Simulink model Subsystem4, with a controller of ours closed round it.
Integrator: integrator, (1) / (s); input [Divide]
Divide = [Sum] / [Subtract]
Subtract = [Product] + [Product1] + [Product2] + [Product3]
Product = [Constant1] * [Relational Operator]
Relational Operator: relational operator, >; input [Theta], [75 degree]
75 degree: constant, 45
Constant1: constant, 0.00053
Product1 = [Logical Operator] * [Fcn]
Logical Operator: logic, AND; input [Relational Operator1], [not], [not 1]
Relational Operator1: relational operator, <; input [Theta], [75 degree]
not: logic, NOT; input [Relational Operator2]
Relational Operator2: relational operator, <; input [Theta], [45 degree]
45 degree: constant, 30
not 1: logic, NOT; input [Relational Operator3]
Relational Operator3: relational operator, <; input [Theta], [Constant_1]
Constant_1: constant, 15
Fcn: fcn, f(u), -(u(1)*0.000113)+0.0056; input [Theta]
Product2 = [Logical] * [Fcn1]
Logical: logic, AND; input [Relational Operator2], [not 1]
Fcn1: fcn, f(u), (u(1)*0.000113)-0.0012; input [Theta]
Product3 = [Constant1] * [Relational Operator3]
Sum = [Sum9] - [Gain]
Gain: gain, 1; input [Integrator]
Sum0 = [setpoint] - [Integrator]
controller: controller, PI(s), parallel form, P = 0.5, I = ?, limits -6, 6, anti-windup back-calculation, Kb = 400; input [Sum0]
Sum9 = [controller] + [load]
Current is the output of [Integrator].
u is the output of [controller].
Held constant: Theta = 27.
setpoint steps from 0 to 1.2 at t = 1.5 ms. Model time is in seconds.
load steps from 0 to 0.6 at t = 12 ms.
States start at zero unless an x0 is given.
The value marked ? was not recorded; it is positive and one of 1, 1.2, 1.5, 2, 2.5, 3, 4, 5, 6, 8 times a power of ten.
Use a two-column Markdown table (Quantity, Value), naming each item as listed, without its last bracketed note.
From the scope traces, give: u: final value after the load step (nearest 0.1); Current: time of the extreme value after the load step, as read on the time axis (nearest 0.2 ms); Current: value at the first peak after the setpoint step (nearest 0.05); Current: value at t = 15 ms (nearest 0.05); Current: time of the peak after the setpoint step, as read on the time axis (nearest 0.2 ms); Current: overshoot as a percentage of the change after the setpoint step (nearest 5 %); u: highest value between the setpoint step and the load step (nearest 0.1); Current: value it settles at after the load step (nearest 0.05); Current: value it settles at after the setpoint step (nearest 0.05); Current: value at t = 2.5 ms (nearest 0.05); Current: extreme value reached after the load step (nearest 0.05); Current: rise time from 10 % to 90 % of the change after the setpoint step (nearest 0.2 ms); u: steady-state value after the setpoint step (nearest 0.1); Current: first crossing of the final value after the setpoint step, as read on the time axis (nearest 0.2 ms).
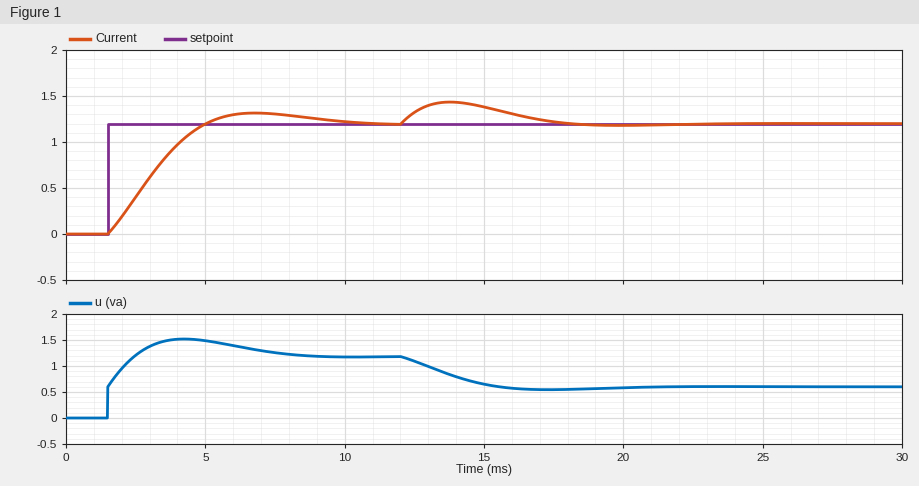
| Quantity | Value |
|---|---|
| u: final value after the load step | 0.6 |
| Current: time of the extreme value after the load step, as read on the time axis | 13.8 ms |
| Current: value at the first peak after the setpoint step | 1.30 |
| Current: value at t = 15 ms | 1.40 |
| Current: time of the peak after the setpoint step, as read on the time axis | 6.8 ms |
| Current: overshoot as a percentage of the change after the setpoint step | 10 % |
| u: highest value between the setpoint step and the load step | 1.5 |
| Current: value it settles at after the load step | 1.20 |
| Current: value it settles at after the setpoint step | 1.20 |
| Current: value at t = 2.5 ms | 0.40 |
| Current: extreme value reached after the load step | 1.45 |
| Current: rise time from 10 % to 90 % of the change after the setpoint step | 2.6 ms |
| u: steady-state value after the setpoint step | 1.2 |
| Current: first crossing of the final value after the setpoint step, as read on the time axis | 5.0 ms |
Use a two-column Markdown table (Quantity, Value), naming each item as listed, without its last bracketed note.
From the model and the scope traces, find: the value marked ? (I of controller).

| Quantity | Value |
|---|---|
| the value marked ? | 800 |
